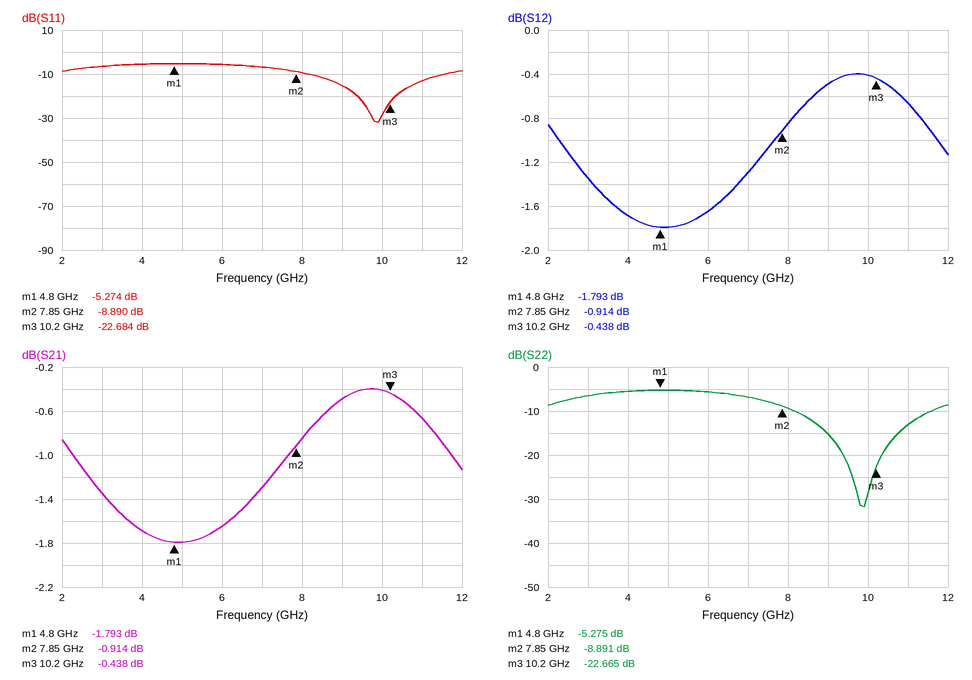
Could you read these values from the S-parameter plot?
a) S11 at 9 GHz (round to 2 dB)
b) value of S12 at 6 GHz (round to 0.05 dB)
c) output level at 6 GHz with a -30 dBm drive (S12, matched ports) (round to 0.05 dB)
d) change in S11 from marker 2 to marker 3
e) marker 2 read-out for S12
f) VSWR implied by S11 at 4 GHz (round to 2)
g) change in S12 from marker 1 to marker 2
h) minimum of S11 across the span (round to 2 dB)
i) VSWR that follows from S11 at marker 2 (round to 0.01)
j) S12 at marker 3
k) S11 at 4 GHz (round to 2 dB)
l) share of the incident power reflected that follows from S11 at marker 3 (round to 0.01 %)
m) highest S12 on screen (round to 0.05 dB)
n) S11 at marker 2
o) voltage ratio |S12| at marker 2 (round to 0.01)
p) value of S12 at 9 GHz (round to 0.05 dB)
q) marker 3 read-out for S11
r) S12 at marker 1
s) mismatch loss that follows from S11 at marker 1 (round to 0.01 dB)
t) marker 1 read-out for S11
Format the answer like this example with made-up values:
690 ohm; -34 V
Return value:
-16 dB; -1.65 dB; -31.65 dBm; -13.794 dB; -0.914 dB; 4; 0.879 dB; -32 dB; 2.12; -0.438 dB; -6 dB; 0.54 %; -0.40 dB; -8.890 dB; 0.90; -0.50 dB; -22.684 dB; -1.793 dB; 1.53 dB; -5.274 dB
